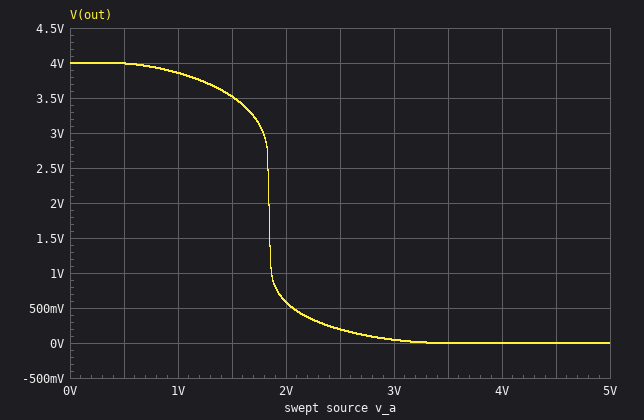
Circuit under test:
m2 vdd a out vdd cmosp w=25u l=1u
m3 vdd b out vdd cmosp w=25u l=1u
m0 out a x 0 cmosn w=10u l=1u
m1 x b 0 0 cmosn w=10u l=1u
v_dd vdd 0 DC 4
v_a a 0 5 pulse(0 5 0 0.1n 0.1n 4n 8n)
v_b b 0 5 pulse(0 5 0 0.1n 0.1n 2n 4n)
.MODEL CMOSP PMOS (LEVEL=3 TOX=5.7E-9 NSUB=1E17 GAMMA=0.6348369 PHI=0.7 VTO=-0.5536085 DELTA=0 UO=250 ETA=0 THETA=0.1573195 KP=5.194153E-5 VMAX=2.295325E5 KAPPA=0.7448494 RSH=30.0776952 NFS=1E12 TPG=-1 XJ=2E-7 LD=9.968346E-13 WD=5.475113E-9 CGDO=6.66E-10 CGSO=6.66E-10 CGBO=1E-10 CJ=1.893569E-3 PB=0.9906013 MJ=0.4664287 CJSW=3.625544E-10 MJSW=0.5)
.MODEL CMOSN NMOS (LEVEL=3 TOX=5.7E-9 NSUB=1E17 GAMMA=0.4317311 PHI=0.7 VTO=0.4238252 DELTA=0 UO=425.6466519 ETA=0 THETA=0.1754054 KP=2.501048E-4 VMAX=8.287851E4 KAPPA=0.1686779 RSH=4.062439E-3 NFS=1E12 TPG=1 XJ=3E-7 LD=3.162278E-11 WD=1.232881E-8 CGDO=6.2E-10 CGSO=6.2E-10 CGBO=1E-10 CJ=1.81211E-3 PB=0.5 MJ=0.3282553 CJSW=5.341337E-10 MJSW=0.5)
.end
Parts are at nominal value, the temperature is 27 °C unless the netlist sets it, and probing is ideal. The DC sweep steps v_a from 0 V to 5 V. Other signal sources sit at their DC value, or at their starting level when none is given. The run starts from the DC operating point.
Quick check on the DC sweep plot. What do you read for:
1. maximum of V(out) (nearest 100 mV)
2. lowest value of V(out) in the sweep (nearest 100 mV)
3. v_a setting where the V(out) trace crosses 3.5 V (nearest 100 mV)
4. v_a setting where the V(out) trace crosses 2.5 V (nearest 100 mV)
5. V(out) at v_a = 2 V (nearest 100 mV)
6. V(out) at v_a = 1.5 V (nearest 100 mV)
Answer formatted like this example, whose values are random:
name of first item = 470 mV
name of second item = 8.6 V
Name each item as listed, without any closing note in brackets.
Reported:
maximum of V(out) = 4.0 V
lowest value of V(out) in the sweep = 0 V
v_a setting where the V(out) trace crosses 3.5 V = 1.5 V
v_a setting where the V(out) trace crosses 2.5 V = 1.8 V
V(out) at v_a = 2 V = 600 mV
V(out) at v_a = 1.5 V = 3.5 V
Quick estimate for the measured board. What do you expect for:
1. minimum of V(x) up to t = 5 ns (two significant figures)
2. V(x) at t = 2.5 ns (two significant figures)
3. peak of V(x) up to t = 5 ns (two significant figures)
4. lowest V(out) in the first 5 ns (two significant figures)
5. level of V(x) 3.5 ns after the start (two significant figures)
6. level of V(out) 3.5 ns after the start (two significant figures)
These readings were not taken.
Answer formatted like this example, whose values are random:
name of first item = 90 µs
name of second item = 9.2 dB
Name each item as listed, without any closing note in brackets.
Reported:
minimum of V(x) up to t = 5 ns = -630 mV
V(x) at t = 2.5 ns = 3.7 V
peak of V(x) up to t = 5 ns = 4.1 V
lowest V(out) in the first 5 ns = -610 mV
level of V(x) 3.5 ns after the start = 4.0 V
level of V(out) 3.5 ns after the start = 4.0 V
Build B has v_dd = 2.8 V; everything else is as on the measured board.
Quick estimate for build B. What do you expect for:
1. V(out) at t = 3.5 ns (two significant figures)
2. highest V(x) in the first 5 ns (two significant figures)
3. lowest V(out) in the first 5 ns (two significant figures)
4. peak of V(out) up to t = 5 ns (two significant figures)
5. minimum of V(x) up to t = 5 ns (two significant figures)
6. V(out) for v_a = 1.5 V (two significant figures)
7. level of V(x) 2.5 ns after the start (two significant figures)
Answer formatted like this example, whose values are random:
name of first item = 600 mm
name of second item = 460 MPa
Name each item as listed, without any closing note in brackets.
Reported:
V(out) at t = 3.5 ns = 2.8 V
highest V(x) in the first 5 ns = 3.1 V
lowest V(out) in the first 5 ns = -670 mV
peak of V(out) up to t = 5 ns = 3.5 V
minimum of V(x) up to t = 5 ns = -650 mV
V(out) for v_a = 1.5 V = 190 mV
level of V(x) 2.5 ns after the start = 2.4 V
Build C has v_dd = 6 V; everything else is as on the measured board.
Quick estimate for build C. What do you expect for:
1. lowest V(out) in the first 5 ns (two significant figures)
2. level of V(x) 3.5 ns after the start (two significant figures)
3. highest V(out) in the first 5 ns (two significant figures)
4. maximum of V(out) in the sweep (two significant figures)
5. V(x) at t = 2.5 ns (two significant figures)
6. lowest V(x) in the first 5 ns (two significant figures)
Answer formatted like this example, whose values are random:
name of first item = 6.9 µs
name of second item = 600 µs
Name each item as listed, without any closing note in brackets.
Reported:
lowest V(out) in the first 5 ns = -170 mV
level of V(x) 3.5 ns after the start = 4.1 V
highest V(out) in the first 5 ns = 6.7 V
maximum of V(out) in the sweep = 6.0 V
V(x) at t = 2.5 ns = 4.0 V
lowest V(x) in the first 5 ns = -320 mV
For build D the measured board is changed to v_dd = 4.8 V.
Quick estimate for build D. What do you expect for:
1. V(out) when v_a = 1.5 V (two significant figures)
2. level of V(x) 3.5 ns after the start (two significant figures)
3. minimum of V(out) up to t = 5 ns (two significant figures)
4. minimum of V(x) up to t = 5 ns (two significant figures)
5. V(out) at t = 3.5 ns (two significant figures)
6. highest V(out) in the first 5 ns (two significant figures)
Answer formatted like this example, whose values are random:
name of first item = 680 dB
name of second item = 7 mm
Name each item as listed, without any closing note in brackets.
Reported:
V(out) when v_a = 1.5 V = 4.4 V
level of V(x) 3.5 ns after the start = 4.1 V
minimum of V(out) up to t = 5 ns = -430 mV
minimum of V(x) up to t = 5 ns = -500 mV
V(out) at t = 3.5 ns = 4.8 V
highest V(out) in the first 5 ns = 5.5 V
